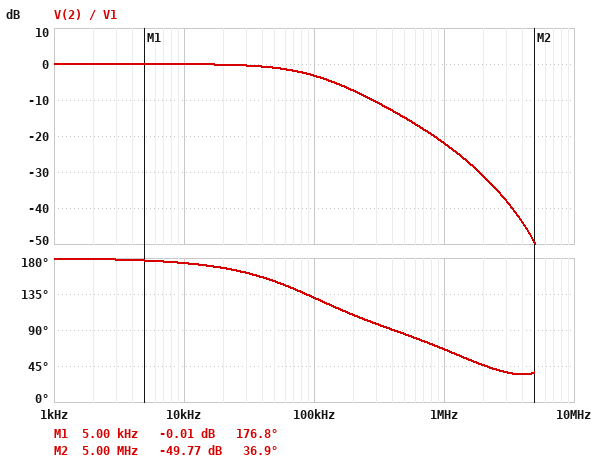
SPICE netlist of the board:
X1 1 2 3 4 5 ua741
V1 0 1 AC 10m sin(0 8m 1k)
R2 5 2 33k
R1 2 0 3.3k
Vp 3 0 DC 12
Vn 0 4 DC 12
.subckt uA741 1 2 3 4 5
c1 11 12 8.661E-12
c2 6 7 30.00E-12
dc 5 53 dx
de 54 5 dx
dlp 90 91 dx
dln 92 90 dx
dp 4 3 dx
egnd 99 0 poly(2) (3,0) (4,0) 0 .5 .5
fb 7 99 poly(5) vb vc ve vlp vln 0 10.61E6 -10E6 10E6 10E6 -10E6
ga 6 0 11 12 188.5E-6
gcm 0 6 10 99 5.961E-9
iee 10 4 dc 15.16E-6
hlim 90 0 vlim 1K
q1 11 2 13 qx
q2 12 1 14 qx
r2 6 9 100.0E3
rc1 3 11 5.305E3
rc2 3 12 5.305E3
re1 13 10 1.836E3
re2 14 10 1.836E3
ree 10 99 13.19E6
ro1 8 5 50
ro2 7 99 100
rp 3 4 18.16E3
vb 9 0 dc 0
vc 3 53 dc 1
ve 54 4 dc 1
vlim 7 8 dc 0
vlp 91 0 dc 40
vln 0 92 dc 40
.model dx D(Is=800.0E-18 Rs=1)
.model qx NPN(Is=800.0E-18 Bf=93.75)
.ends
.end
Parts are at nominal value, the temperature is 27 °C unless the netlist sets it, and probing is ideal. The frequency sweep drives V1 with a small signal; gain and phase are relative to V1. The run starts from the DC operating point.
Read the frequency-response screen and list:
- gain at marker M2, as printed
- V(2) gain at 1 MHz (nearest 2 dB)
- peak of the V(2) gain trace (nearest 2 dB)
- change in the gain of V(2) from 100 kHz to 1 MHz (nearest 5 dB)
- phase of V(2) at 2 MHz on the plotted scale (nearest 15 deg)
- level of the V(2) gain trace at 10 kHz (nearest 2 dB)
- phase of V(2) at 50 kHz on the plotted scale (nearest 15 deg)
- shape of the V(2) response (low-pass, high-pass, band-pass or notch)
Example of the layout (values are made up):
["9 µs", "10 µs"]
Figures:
["-49.77 dB", "-22 dB", "0 dB", "-20 dB", "45 deg", "0 dB", "150 deg", "low-pass"]
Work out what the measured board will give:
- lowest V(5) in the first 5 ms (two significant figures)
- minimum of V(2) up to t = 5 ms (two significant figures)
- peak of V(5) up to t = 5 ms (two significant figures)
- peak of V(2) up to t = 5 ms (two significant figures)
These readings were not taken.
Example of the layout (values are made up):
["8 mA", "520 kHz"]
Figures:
["-85 mV", "-8.0 mV", "91 mV", "8.0 mV"]
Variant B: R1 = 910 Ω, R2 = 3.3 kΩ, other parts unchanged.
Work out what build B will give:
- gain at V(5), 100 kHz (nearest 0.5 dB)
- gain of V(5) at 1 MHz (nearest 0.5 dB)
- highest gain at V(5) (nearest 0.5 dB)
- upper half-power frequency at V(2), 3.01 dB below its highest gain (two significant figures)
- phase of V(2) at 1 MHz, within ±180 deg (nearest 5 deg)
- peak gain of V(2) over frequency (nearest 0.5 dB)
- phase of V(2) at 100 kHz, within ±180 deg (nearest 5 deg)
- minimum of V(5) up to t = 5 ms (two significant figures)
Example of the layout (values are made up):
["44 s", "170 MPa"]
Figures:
["12.5 dB", "-0.5 dB", "13.5 dB", "240 kHz", "70 deg", "0 dB", "155 deg", "-37 mV"]
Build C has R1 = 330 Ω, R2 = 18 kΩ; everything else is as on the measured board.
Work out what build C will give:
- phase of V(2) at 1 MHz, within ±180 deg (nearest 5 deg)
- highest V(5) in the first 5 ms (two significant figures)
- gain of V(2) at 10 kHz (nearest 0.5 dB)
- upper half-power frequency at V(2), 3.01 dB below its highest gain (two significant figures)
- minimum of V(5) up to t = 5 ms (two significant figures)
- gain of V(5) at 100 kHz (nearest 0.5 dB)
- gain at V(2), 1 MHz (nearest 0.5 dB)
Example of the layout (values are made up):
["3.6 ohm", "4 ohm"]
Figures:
["60 deg", "450 mV", "-1.0 dB", "18 kHz", "-440 mV", "20.0 dB", "-36.0 dB"]
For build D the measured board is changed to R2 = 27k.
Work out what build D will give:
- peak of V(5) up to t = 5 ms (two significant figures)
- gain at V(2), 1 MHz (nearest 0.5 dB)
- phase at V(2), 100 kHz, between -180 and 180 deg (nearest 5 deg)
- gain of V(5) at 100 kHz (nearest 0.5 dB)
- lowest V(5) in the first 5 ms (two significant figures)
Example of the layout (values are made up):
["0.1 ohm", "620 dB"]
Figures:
["76 mV", "-20.5 dB", "135 deg", "17.0 dB", "-71 mV"]
